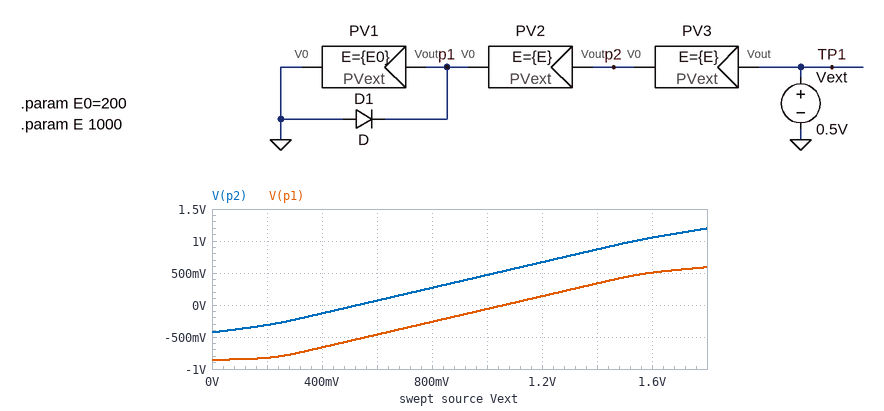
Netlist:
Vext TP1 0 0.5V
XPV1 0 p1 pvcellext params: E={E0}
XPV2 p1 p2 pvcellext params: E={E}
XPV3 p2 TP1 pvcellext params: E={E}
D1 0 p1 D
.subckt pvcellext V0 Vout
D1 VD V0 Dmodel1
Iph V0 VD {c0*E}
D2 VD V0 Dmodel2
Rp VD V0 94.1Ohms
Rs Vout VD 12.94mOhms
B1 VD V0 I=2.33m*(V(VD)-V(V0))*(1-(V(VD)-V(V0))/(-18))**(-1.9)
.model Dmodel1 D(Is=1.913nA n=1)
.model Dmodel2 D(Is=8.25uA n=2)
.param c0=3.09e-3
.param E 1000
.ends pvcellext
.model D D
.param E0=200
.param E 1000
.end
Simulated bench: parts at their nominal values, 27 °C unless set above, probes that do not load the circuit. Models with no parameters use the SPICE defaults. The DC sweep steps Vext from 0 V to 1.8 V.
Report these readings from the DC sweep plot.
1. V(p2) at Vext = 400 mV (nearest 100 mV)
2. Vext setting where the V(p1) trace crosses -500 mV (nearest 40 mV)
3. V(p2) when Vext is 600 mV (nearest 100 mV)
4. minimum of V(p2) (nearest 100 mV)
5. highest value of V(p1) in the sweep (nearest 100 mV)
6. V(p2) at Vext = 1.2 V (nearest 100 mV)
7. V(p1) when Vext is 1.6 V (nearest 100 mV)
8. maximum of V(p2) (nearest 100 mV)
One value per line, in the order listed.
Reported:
-100 mV
560 mV
100 mV
-400 mV
600 mV
700 mV
500 mV
1.2 V
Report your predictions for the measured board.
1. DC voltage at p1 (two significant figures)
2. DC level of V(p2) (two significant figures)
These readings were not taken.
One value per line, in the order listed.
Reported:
-560 mV
-31 mV
